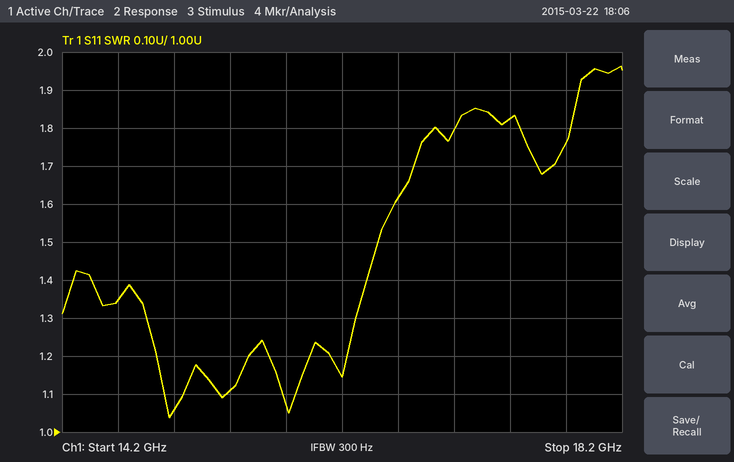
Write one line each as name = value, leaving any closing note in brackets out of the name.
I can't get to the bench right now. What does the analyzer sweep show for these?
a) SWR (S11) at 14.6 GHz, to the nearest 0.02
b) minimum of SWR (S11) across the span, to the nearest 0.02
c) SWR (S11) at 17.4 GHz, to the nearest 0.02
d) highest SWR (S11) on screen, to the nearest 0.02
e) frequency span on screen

SWR (S11) at 14.6 GHz, to the nearest 0.02 = 1.34
minimum of SWR (S11) across the span, to the nearest 0.02 = 1.04
SWR (S11) at 17.4 GHz, to the nearest 0.02 = 1.82
highest SWR (S11) on screen, to the nearest 0.02 = 1.96
frequency span on screen = 4 GHz
